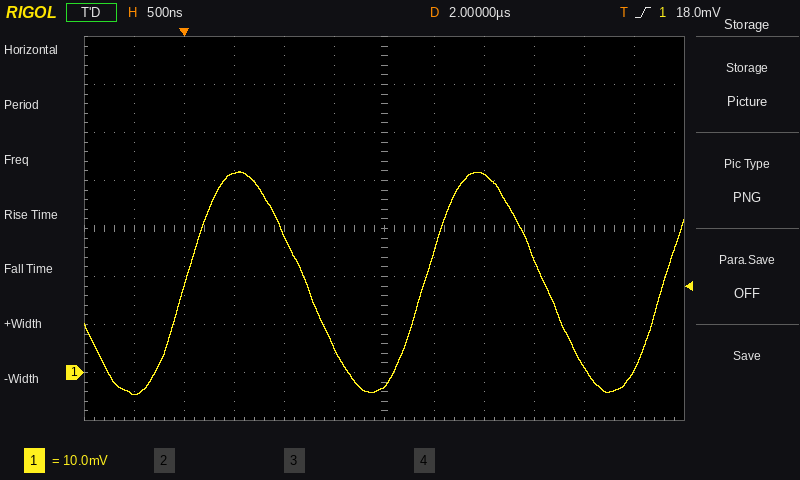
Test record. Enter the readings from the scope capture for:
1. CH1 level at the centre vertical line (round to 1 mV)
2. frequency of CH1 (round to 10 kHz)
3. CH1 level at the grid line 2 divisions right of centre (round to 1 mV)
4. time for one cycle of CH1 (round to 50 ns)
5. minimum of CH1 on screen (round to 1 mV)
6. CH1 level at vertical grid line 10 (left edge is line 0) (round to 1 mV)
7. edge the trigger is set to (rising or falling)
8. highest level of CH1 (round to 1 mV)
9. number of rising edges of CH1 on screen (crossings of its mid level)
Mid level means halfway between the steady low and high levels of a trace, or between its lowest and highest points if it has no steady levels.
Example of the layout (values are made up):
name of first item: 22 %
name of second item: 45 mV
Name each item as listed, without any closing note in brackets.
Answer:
CH1 level at the centre vertical line: -3 mV
frequency of CH1: 420 kHz
CH1 level at the grid line 2 divisions right of centre: 41 mV
time for one cycle of CH1: 2.40 µs
minimum of CH1 on screen: -5 mV
CH1 level at vertical grid line 10 (left edge is line 0): 1 mV
edge the trigger is set to: rising
highest level of CH1: 42 mV
number of rising edges of CH1 on screen: 3
